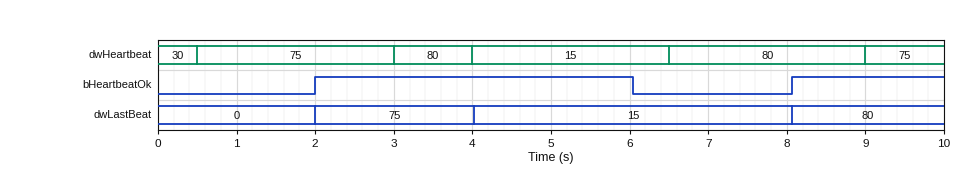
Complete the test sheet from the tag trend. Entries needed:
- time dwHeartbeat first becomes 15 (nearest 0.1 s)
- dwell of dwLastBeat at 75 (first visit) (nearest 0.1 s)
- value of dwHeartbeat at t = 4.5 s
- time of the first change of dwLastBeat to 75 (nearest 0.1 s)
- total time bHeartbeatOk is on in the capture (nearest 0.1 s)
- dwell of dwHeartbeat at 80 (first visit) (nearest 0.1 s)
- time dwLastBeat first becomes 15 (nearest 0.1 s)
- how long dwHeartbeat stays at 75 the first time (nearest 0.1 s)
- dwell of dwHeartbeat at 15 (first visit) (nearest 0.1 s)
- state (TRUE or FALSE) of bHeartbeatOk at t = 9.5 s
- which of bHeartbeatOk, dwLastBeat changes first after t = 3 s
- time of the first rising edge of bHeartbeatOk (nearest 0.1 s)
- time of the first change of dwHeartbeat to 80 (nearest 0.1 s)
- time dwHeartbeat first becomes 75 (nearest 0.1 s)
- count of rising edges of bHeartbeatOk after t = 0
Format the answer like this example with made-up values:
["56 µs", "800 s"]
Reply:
["4.0 s", "2.0 s", "15", "2.0 s", "6.0 s", "1.0 s", "4.0 s", "2.5 s", "2.5 s", "TRUE", "dwLastBeat", "2.0 s", "3.0 s", "0.5 s", "2"]
